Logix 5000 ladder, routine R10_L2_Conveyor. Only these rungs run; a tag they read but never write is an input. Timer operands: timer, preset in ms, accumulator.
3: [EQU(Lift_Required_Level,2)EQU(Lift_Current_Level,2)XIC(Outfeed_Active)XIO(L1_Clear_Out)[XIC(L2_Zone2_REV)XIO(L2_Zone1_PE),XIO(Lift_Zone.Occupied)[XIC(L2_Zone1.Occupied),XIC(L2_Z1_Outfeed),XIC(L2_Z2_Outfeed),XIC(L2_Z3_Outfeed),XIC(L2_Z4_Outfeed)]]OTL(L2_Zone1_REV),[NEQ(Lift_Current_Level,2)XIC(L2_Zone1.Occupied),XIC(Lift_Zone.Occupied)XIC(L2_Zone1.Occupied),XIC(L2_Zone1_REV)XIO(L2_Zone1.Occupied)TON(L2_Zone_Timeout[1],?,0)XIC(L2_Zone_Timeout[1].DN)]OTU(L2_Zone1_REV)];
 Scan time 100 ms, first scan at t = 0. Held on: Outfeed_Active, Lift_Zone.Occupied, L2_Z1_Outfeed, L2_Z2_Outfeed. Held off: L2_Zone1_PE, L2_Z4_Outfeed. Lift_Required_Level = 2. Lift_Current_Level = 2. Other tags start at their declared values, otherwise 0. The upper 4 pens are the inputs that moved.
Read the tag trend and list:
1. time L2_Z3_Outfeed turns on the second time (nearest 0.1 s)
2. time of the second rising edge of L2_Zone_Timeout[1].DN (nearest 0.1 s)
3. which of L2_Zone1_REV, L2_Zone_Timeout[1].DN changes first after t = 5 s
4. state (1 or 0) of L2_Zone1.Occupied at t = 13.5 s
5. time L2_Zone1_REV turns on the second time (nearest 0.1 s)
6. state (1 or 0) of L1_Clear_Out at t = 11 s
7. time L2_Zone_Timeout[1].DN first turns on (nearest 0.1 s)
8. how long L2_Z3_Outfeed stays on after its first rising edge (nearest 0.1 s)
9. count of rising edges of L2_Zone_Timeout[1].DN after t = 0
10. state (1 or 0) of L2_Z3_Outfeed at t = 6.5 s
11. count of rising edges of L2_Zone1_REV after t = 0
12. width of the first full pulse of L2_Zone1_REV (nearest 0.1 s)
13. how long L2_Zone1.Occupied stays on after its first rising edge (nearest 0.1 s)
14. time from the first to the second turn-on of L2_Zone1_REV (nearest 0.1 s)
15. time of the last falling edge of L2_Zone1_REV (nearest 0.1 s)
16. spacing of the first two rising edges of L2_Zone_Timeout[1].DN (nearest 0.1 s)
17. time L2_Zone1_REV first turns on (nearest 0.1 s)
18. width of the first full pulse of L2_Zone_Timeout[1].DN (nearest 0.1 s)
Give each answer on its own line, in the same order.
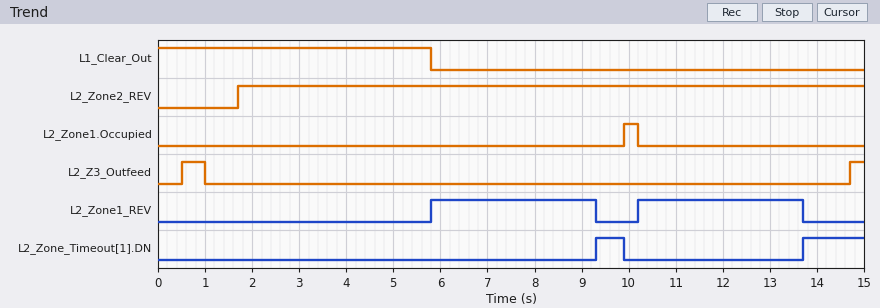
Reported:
14.7 s
13.7 s
L2_Zone1_REV
0
10.2 s
0
9.3 s
0.5 s
2
0
2
3.5 s
0.3 s
4.4 s
13.7 s
4.4 s
5.8 s
0.6 s
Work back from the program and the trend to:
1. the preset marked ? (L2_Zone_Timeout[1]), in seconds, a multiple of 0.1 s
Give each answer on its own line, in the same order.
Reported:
3.5 s
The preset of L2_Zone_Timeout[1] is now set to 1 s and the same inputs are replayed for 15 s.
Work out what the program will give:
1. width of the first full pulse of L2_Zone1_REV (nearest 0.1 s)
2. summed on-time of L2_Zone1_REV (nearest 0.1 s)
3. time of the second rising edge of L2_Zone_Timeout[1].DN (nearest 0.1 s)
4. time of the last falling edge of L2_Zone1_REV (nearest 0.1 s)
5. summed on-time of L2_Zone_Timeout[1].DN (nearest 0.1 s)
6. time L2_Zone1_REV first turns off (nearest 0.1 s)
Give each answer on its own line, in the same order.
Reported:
1.0 s
2.0 s
11.2 s
11.2 s
6.9 s
6.8 s
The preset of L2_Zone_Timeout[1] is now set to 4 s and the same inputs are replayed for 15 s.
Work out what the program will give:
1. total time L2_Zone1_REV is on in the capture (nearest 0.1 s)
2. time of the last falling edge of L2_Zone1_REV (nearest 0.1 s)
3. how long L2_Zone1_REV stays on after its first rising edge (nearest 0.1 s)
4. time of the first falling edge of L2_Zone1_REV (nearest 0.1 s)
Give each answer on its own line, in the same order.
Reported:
8.0 s
14.2 s
4.0 s
9.8 s
